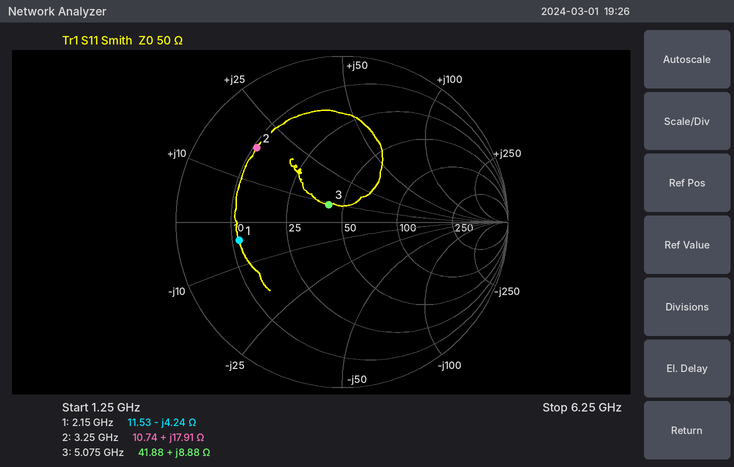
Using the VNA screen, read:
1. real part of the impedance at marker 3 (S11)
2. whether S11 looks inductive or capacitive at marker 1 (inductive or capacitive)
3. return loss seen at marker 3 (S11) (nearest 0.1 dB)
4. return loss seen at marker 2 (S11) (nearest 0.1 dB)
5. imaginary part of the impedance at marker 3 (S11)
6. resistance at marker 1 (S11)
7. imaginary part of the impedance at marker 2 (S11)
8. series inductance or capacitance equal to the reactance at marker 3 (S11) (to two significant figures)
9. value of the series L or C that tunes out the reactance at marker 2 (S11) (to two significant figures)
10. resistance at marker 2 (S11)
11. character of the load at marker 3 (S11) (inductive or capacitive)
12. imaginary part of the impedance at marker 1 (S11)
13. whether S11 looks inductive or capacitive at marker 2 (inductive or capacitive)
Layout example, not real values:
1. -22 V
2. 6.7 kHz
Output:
1. 41.88 Ω
2. capacitive
3. 17.7 dB
4. 3.3 dB
5. +8.88 Ω
6. 11.53 Ω
7. +17.91 Ω
8. 280 pH
9. 2.7 pF
10. 10.74 Ω
11. inductive
12. -4.24 Ω
13. inductive
